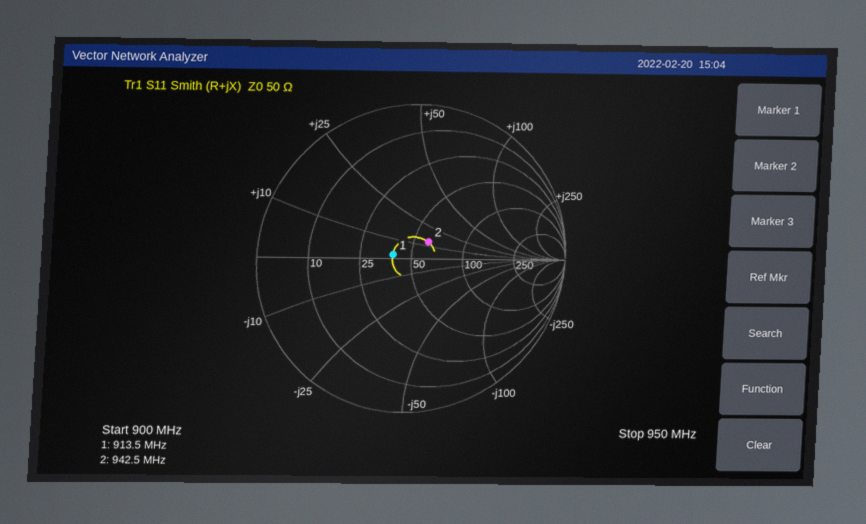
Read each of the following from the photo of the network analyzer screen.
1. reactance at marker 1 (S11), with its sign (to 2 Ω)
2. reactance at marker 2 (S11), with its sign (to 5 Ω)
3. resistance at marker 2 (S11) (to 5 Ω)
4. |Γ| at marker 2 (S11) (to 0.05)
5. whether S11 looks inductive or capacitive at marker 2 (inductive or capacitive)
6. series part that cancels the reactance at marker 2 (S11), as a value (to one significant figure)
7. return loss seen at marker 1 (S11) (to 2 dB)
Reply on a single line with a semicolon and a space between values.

+2 Ω; +15 Ω; 60 Ω; 0.15; inductive; 10 pF; 18 dB
